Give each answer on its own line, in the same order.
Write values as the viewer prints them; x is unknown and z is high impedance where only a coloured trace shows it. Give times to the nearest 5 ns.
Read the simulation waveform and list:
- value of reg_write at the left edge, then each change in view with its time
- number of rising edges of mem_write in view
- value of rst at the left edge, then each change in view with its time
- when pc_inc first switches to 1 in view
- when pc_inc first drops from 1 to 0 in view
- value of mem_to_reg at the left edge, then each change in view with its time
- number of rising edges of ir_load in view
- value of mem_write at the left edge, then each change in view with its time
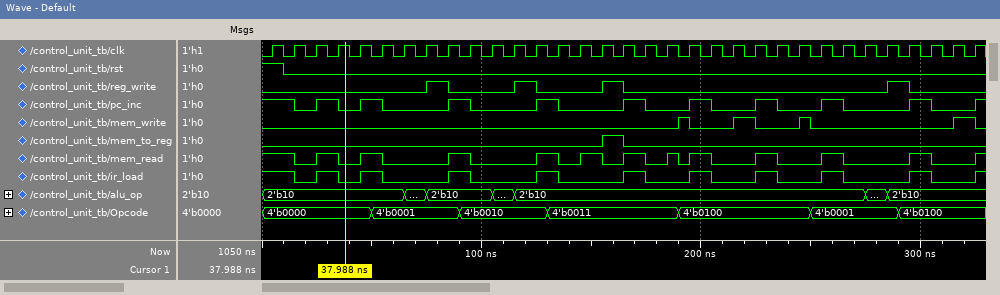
0, 1 at 75 ns, 0 at 85 ns, 1 at 115 ns, 0 at 125 ns, 1 at 155 ns, 0 at 165 ns, 1 at 285 ns, 0 at 295 ns
4
1, 0 at 10 ns
25 ns
15 ns
0, 1 at 155 ns, 0 at 165 ns
10
0, 1 at 190 ns, 0 at 195 ns, 1 at 215 ns, 0 at 225 ns, 1 at 245 ns, 0 at 250 ns, 1 at 315 ns, 0 at 325 ns
